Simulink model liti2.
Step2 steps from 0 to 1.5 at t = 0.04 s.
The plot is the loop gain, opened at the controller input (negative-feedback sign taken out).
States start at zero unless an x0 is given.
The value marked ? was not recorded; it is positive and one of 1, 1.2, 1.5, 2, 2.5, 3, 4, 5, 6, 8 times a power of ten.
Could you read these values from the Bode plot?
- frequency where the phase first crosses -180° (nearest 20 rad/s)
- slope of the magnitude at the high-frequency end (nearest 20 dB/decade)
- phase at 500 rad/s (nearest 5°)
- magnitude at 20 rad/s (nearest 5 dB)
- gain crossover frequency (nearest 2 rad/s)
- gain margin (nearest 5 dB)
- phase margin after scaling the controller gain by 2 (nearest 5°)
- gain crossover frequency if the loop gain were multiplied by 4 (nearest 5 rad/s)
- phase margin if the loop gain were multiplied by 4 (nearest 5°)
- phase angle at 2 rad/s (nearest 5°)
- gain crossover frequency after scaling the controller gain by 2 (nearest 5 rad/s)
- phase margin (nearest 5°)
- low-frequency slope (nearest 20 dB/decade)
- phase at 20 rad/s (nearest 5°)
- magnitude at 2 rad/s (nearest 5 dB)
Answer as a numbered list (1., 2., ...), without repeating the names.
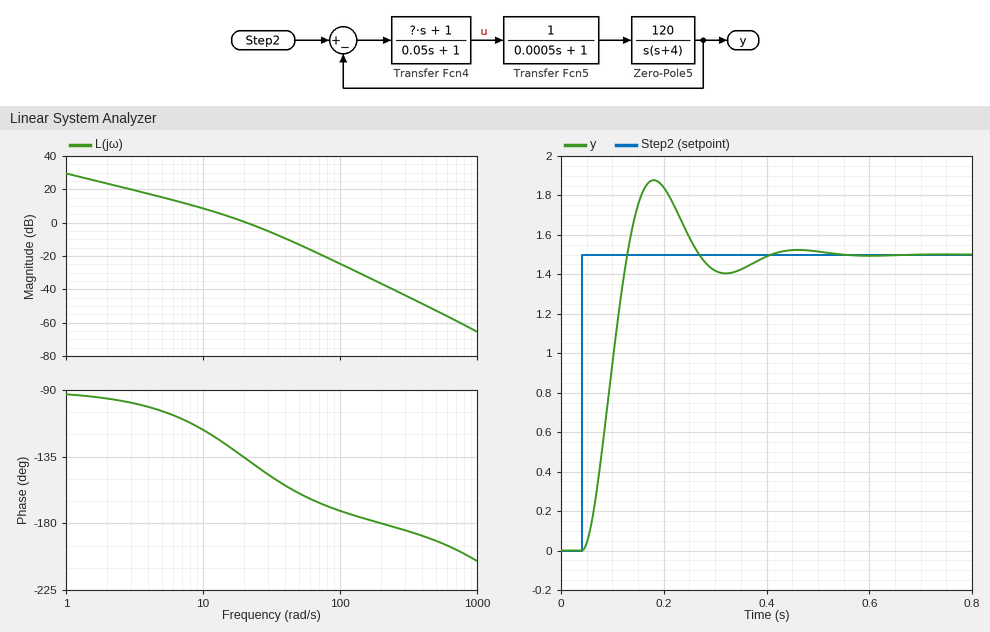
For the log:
1. 200 rad/s
2. -40 dB/decade
3. -190°
4. 0 dB
5. 20 rad/s
6. 35 dB
7. 30°
8. 45 rad/s
9. 20°
10. -95°
11. 30 rad/s
12. 45°
13. -20 dB/decade
14. -135°
15. 25 dB
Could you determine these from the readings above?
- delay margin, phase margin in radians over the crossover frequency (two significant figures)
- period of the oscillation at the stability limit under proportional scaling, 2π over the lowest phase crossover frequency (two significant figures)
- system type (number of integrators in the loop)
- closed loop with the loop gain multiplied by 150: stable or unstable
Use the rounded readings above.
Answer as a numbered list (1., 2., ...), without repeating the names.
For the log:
1. 0.039 s
2. 0.031 s
3. 1
4. unstable
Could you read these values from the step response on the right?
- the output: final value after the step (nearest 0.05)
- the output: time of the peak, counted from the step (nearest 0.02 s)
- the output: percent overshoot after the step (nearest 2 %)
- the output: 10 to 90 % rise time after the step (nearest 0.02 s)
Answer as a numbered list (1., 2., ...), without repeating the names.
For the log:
1. 1.50
2. 0.14 s
3. 26 %
4. 0.06 s
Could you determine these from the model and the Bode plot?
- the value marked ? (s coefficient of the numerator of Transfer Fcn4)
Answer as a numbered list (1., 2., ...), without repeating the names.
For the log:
1. 0.25
